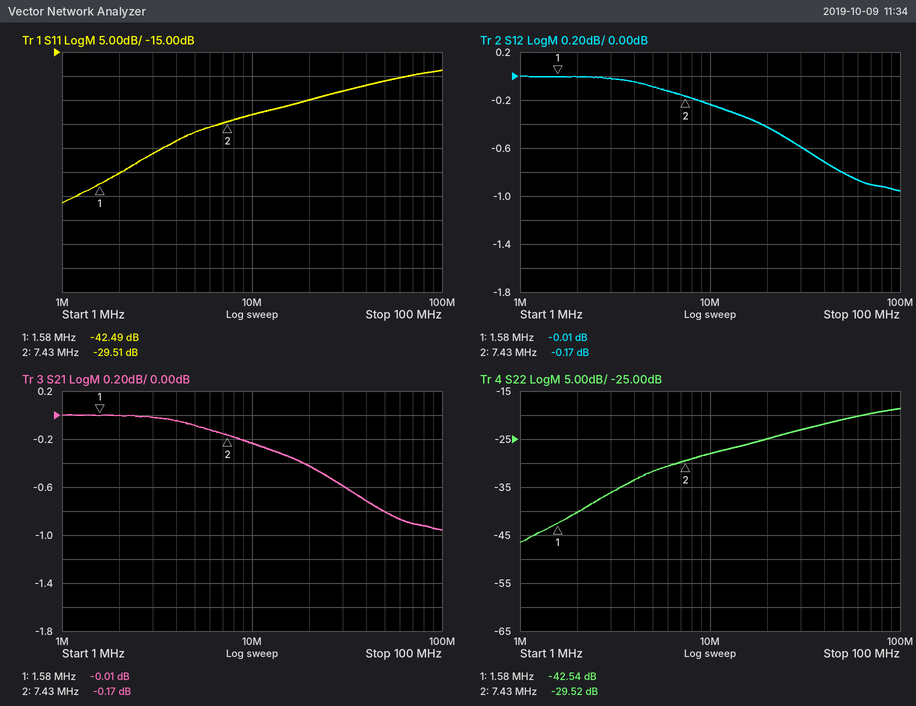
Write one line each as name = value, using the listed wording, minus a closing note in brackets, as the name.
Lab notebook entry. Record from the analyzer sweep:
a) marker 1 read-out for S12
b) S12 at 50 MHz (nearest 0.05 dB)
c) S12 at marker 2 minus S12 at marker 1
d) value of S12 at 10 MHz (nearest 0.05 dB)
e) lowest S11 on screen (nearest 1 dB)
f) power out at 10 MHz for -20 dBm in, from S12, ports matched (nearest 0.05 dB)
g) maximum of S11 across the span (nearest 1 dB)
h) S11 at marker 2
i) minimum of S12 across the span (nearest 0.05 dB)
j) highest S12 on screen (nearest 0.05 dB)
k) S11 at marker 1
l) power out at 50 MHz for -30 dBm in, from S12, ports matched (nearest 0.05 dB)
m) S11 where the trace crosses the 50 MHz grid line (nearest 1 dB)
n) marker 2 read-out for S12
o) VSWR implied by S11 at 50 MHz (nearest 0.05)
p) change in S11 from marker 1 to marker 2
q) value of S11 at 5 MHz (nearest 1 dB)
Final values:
marker 1 read-out for S12 = -0.01 dB
S12 at 50 MHz = -0.80 dB
S12 at marker 2 minus S12 at marker 1 = -0.16 dB
value of S12 at 10 MHz = -0.25 dB
lowest S11 on screen = -46 dB
power out at 10 MHz for -20 dBm in, from S12, ports matched = -20.25 dBm
maximum of S11 across the span = -19 dB
S11 at marker 2 = -29.51 dB
minimum of S12 across the span = -0.95 dB
highest S12 on screen = 0.00 dB
S11 at marker 1 = -42.49 dB
power out at 50 MHz for -30 dBm in, from S12, ports matched = -30.80 dBm
S11 where the trace crosses the 50 MHz grid line = -21 dB
marker 2 read-out for S12 = -0.17 dB
VSWR implied by S11 at 50 MHz = 1.20
change in S11 from marker 1 to marker 2 = 12.98 dB
value of S11 at 5 MHz = -32 dB
